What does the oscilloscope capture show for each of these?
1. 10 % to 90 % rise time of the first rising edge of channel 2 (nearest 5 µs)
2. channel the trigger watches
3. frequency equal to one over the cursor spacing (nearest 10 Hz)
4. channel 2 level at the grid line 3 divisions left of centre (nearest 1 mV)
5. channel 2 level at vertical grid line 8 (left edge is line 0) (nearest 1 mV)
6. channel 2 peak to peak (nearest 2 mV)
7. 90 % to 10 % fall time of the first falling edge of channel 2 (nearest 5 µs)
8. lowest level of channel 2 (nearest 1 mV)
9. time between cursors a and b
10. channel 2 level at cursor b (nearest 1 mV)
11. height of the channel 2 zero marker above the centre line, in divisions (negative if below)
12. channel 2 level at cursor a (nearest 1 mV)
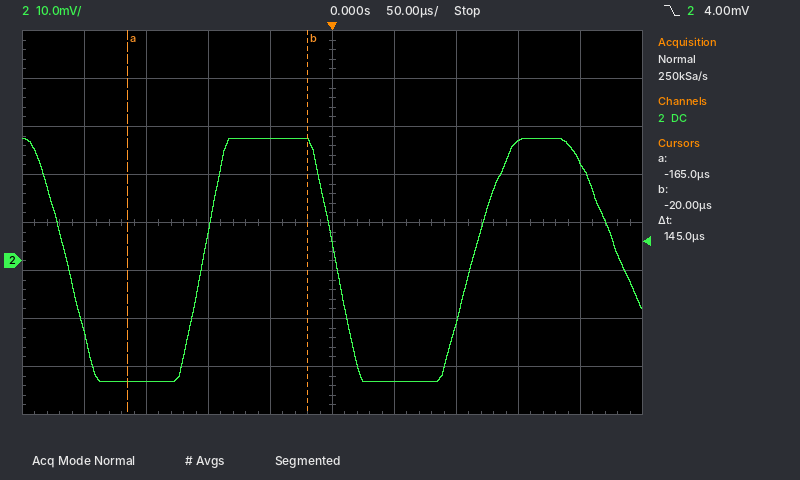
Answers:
30 µs
channel 2
6.90 kHz
-25 mV
25 mV
50 mV
40 µs
-25 mV
145 µs
25 mV
-0.8 div
-25 mV
